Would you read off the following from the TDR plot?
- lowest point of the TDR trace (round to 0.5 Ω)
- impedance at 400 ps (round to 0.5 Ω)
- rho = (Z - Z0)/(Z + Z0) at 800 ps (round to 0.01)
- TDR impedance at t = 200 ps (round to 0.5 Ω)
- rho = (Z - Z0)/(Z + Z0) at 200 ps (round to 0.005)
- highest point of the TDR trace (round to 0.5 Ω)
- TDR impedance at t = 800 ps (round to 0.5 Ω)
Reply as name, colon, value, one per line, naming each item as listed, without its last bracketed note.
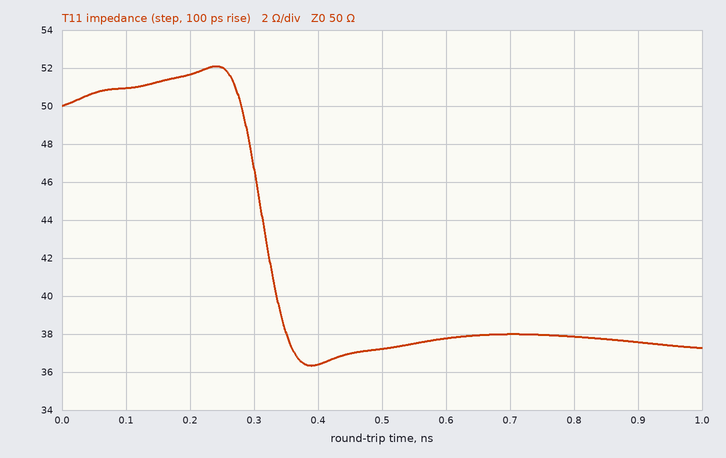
lowest point of the TDR trace: 36.5 Ω
impedance at 400 ps: 36.5 Ω
rho = (Z - Z0)/(Z + Z0) at 800 ps: -0.14
TDR impedance at t = 200 ps: 51.5 Ω
rho = (Z - Z0)/(Z + Z0) at 200 ps: +0.015
highest point of the TDR trace: 52.0 Ω
TDR impedance at t = 800 ps: 38.0 Ω
